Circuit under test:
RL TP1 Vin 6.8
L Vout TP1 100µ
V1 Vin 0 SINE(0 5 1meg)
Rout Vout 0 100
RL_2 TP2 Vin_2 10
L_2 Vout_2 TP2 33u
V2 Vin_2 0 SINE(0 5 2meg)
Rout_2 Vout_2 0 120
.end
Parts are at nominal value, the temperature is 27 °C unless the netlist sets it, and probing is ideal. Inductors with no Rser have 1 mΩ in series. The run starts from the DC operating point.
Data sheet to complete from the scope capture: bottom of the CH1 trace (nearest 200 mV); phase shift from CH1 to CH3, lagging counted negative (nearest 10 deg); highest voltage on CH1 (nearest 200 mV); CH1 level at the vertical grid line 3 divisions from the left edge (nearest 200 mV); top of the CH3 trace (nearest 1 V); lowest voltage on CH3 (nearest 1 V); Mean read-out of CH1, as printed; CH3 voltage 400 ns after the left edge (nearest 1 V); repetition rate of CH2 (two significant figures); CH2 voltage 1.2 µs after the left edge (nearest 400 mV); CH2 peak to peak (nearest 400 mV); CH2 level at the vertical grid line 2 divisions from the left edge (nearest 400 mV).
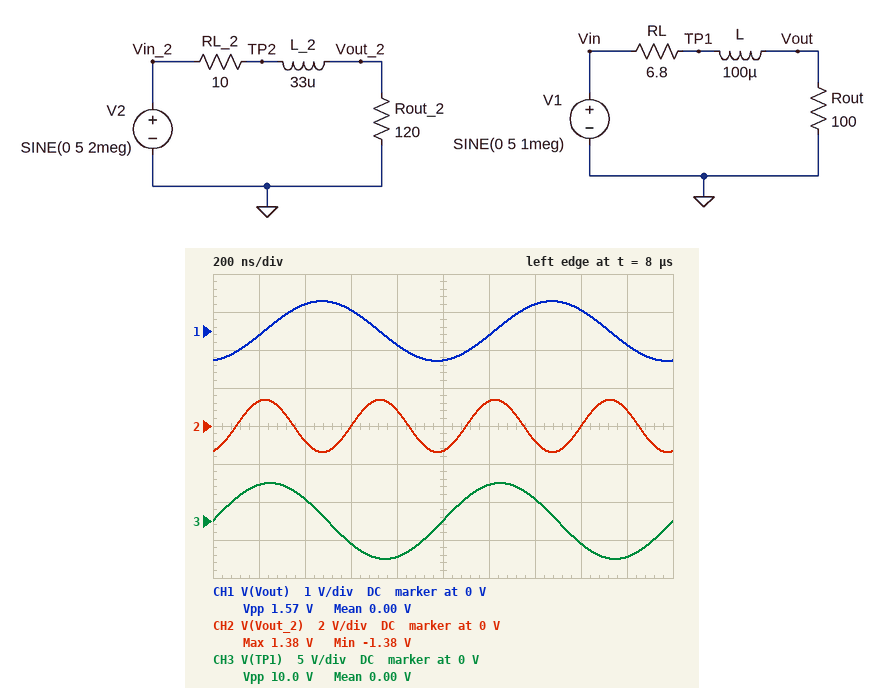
-800 mV
80 deg
800 mV
600 mV
5 V
-5 V
0.00 V
3 V
2.0 MHz
1.2 V
2.8 V
-800 mV
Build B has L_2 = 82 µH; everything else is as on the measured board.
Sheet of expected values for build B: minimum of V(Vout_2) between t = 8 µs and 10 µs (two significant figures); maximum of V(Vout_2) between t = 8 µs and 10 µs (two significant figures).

-580 mV
580 mV
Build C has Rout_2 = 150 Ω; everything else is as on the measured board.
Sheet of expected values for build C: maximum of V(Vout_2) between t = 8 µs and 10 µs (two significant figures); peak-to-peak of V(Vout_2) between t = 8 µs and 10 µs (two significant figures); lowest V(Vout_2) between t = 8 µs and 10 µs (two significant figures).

1.7 V
3.4 V
-1.7 V
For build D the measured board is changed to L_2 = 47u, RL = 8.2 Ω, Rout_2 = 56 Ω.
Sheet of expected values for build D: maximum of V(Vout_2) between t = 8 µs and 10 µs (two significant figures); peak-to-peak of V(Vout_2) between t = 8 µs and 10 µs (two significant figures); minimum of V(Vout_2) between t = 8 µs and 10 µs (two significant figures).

470 mV
940 mV
-470 mV
